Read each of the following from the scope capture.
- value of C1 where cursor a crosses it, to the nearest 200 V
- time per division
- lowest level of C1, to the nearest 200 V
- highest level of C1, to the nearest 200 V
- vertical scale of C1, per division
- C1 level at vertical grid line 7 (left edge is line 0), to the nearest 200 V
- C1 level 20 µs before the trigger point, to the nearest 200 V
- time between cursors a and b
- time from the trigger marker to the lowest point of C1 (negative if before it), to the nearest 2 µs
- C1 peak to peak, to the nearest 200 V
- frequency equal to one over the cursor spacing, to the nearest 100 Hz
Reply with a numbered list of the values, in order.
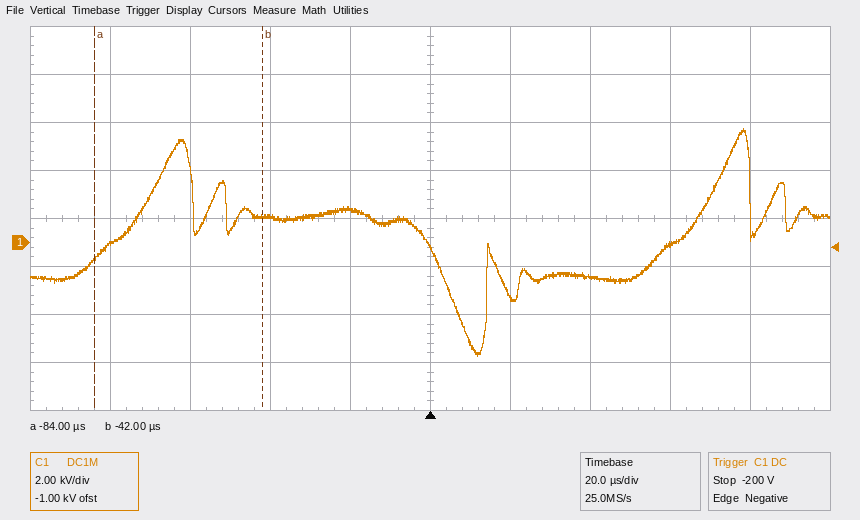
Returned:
1. -600 V
2. 20 µs
3. -4.8 kV
4. 4.8 kV
5. 2 kV
6. -1.4 kV
7. 1.4 kV
8. 42 µs
9. +12 µs
10. 9.6 kV
11. 23.8 kHz
